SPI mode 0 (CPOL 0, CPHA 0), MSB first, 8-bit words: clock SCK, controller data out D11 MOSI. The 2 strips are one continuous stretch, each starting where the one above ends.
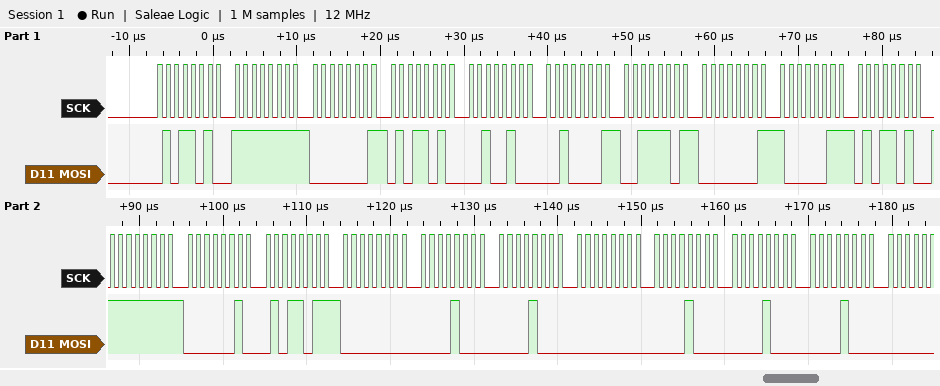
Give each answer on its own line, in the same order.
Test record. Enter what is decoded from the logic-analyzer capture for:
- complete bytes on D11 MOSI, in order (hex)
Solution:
0x5A 0xFF 0x01 0x5A 0x24 0x21 0x3D 0x01 0x83 0x5A 0xFF 0x02 0x5B 0x00 0x08 0x08 0x00 0x08 0x08 0x08
